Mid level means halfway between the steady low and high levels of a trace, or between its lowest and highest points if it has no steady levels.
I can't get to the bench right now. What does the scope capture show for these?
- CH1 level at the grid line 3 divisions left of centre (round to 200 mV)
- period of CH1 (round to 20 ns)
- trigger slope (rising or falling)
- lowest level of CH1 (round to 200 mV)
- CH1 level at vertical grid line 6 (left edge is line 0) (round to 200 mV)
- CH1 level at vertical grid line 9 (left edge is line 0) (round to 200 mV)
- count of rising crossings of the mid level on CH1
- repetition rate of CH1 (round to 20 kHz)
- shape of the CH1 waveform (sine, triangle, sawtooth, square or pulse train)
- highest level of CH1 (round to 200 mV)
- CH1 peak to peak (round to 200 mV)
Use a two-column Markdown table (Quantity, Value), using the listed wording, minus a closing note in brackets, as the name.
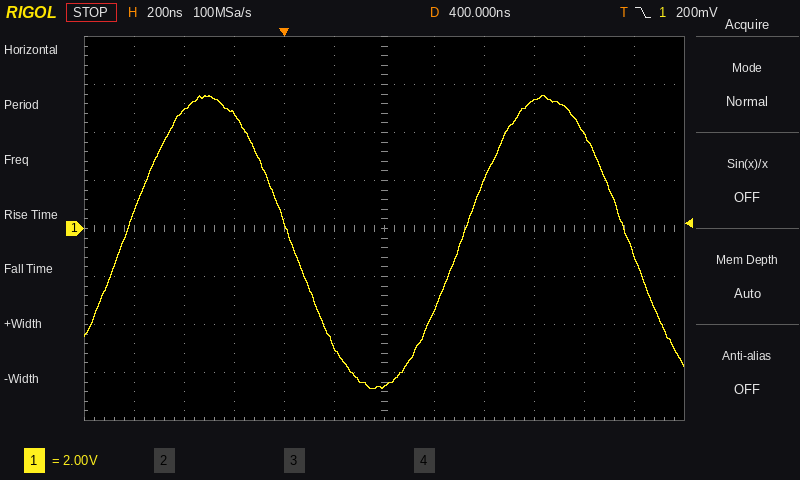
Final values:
| Quantity | Value |
|---|---|
| CH1 level at the grid line 3 divisions left of centre | 4.8 V |
| period of CH1 | 1.36 µs |
| trigger slope | falling |
| lowest level of CH1 | -6.6 V |
| CH1 level at vertical grid line 6 (left edge is line 0) | -6.6 V |
| CH1 level at vertical grid line 9 (left edge is line 0) | 5.4 V |
| count of rising crossings of the mid level on CH1 | 2 |
| repetition rate of CH1 | 740 kHz |
| shape of the CH1 waveform | sine |
| highest level of CH1 | 5.6 V |
| CH1 peak to peak | 12.2 V |
